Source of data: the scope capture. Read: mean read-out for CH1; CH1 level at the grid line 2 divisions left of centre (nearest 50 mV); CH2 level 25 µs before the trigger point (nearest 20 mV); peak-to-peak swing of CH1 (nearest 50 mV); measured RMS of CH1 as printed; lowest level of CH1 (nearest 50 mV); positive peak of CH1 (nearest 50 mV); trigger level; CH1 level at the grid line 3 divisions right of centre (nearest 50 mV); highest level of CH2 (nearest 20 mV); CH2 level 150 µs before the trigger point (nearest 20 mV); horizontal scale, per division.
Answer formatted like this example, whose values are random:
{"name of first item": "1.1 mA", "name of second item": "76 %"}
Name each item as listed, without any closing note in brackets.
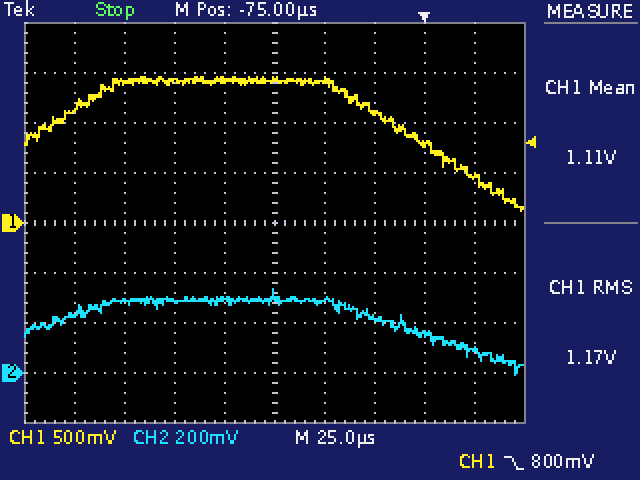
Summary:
{"mean read-out for CH1": "1.11 V", "CH1 level at the grid line 2 divisions left of centre": "1.40 V", "CH2 level 25 µs before the trigger point": "220 mV", "peak-to-peak swing of CH1": "1.35 V", "measured RMS of CH1 as printed": "1.17 V", "lowest level of CH1": "100 mV", "positive peak of CH1": "1.45 V", "trigger level": "800 mV", "CH1 level at the grid line 3 divisions right of centre": "800 mV", "highest level of CH2": "340 mV", "CH2 level 150 µs before the trigger point": "280 mV", "horizontal scale, per division": "25 µs"}
